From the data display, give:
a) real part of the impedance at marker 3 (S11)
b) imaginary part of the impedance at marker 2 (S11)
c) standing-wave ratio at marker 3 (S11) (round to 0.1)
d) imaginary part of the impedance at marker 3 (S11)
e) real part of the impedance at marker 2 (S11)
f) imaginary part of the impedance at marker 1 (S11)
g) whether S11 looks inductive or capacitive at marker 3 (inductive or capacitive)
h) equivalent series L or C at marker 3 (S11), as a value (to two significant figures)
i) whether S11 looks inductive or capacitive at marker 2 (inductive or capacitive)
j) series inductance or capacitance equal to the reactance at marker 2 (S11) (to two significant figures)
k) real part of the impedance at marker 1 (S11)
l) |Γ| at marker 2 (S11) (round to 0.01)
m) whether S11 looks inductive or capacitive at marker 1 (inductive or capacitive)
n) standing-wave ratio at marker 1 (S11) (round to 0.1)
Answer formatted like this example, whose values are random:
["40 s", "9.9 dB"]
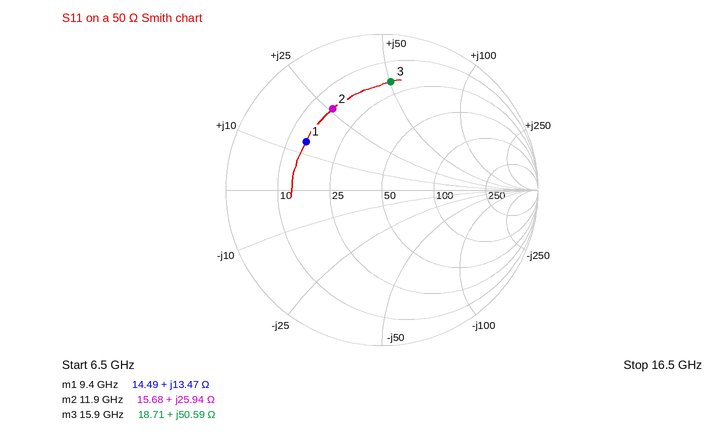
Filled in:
["18.71 Ω", "+25.94 Ω", "5.6", "+50.59 Ω", "15.68 Ω", "+13.47 Ω", "inductive", "510 pH", "inductive", "350 pH", "14.49 Ω", "0.61", "inductive", "3.7"]
